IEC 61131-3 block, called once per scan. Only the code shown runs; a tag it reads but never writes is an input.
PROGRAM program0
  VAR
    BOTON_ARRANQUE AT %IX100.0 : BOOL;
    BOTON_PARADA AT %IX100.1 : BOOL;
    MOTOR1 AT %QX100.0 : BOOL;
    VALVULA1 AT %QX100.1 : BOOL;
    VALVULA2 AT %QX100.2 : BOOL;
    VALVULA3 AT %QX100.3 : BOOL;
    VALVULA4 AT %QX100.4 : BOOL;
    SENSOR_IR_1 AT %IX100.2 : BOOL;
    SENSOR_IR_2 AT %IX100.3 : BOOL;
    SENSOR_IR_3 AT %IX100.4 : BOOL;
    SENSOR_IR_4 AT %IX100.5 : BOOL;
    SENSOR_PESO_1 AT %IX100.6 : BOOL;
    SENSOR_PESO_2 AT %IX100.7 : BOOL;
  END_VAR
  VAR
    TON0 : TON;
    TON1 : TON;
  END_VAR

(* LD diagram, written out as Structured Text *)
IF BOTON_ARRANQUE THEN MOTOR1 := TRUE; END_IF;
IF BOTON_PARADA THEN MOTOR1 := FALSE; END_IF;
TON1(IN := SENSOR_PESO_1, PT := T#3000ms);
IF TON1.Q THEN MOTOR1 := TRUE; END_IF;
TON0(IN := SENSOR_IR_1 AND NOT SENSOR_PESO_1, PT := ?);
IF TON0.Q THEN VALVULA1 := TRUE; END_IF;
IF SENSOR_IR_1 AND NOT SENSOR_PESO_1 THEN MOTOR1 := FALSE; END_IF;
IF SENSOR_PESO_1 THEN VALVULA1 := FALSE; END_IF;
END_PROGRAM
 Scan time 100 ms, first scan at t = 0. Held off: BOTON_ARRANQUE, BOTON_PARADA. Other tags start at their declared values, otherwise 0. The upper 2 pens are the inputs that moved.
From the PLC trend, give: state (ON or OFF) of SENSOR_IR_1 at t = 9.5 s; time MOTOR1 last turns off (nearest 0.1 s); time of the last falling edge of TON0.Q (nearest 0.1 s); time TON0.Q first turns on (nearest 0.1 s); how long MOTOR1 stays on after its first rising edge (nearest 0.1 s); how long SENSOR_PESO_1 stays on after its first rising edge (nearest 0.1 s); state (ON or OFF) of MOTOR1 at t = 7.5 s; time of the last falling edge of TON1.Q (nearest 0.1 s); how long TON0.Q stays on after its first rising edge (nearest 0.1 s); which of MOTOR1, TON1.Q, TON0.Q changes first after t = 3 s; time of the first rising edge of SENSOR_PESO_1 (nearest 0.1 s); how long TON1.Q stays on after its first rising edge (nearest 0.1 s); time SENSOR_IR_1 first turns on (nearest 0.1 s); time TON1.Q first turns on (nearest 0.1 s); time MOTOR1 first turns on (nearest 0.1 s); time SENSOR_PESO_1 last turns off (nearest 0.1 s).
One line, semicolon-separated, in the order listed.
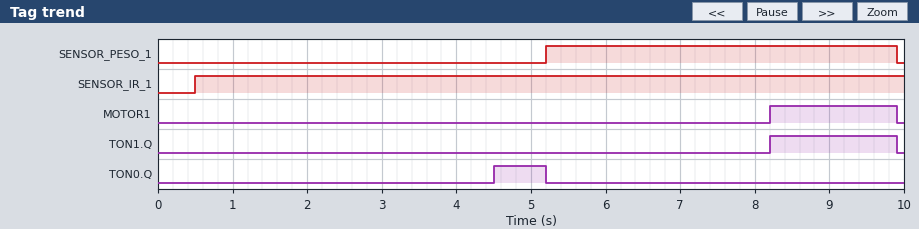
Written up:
ON; 9.9 s; 5.2 s; 4.5 s; 1.7 s; 4.7 s; OFF; 9.9 s; 0.7 s; TON0.Q; 5.2 s; 1.7 s; 0.5 s; 8.2 s; 8.2 s; 9.9 s
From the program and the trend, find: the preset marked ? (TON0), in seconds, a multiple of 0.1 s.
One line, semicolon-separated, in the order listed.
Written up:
4.0 s
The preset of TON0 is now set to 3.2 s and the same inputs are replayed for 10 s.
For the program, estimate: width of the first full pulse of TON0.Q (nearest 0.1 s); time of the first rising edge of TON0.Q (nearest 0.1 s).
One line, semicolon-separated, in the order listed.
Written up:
1.5 s; 3.7 s
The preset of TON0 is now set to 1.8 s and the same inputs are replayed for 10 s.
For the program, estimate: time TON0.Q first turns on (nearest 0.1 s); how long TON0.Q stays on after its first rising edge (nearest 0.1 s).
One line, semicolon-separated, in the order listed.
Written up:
2.3 s; 2.9 s
